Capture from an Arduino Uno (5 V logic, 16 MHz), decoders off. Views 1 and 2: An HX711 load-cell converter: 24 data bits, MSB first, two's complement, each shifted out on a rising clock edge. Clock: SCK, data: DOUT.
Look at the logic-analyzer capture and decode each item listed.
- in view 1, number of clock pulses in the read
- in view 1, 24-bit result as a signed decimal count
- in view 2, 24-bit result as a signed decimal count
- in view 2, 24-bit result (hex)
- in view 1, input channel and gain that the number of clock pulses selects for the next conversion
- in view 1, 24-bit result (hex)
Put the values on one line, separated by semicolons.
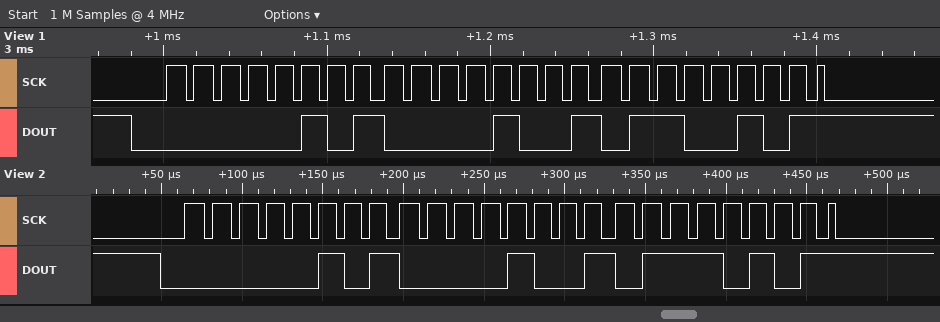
25; 330085; 330101; 0x050975; channel A, gain 128; 0x050965
